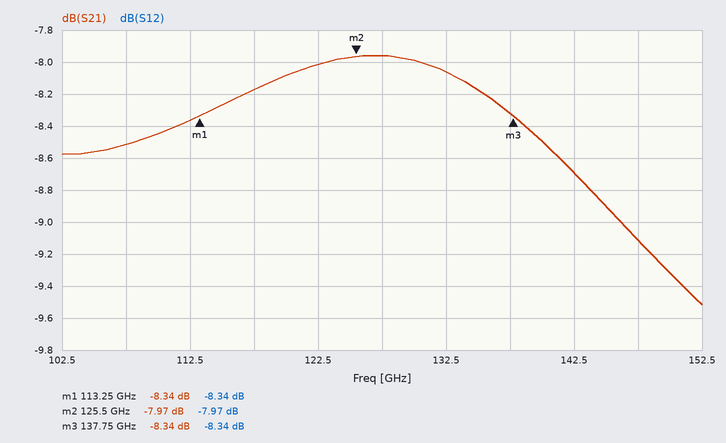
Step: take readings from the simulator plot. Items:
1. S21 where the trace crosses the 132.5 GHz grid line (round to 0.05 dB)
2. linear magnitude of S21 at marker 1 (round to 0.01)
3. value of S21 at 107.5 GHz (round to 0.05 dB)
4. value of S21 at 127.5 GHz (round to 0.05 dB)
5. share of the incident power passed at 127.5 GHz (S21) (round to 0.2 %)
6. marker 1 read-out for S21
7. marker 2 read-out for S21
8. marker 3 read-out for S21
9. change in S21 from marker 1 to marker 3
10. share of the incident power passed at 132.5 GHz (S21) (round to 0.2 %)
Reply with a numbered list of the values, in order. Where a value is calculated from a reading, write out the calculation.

1. -8.05 dB
2. 10^(-8.34/20) ≈ 0.38
3. -8.50 dB
4. -7.95 dB
5. 10^(-7.95/10) ≈ 16.0 %
6. -8.34 dB
7. -7.97 dB
8. -8.34 dB
9. -8.34 − (-8.34) = 0.00 dB
10. 10^(-8.05/10) ≈ 15.7 %, so 15.6 % to the nearest 0.2 %
